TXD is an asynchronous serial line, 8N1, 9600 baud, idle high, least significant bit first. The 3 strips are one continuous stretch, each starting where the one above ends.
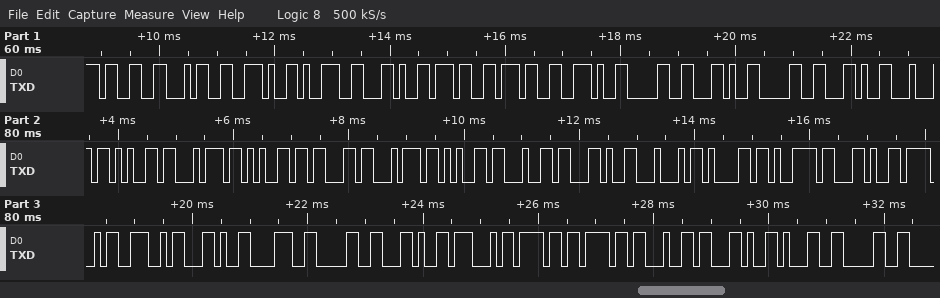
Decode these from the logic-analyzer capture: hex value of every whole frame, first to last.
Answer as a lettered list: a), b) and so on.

a) 33 34 2E 39 2C 37 37 2E 30 2C 30 2C 44 65 74 65 63 74 65 64 2C 44 61 79 2C 4F 4E 2C 38 30 2C 47 6F 6F 64 2C 31 30
